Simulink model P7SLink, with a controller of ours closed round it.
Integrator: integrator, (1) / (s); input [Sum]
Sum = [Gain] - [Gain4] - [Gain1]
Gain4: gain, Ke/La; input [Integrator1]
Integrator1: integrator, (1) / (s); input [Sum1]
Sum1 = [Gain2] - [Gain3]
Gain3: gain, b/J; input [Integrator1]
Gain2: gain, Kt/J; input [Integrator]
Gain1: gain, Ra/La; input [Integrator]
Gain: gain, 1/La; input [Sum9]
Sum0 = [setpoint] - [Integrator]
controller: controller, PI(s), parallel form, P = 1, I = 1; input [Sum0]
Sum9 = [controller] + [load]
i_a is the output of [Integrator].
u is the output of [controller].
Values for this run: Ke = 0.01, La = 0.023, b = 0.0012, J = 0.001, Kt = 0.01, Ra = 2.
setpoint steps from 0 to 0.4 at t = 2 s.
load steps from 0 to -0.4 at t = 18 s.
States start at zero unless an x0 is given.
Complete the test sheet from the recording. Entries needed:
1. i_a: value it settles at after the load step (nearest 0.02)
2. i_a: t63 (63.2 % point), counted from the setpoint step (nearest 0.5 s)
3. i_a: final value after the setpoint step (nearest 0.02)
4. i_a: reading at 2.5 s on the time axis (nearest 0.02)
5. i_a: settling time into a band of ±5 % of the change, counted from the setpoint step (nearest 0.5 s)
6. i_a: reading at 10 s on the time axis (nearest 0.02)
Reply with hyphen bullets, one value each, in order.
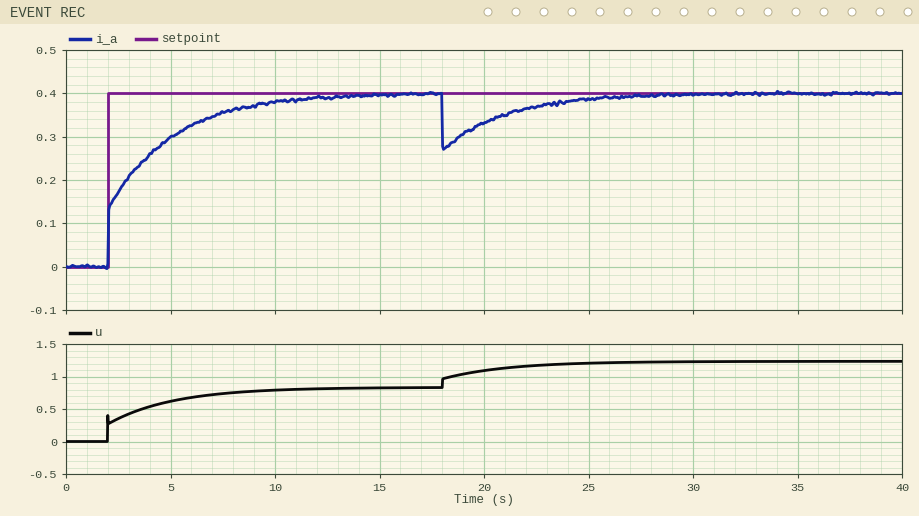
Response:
- 0.40
- 2.0 s
- 0.40
- 0.18
- 8.0 s
- 0.38
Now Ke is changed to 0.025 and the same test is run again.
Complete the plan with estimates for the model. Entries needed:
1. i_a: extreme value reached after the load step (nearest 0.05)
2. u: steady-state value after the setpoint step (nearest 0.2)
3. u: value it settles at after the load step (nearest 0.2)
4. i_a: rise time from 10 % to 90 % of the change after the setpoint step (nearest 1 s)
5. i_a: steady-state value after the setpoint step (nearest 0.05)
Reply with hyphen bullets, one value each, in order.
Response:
- 0.25
- 0.8
- 1.2
- 6 s
- 0.40
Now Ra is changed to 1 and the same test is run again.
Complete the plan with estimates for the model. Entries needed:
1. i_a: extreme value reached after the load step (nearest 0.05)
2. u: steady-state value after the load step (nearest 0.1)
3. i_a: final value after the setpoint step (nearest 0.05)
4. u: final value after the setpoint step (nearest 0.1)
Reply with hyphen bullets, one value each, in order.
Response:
- 0.20
- 0.8
- 0.40
- 0.4
